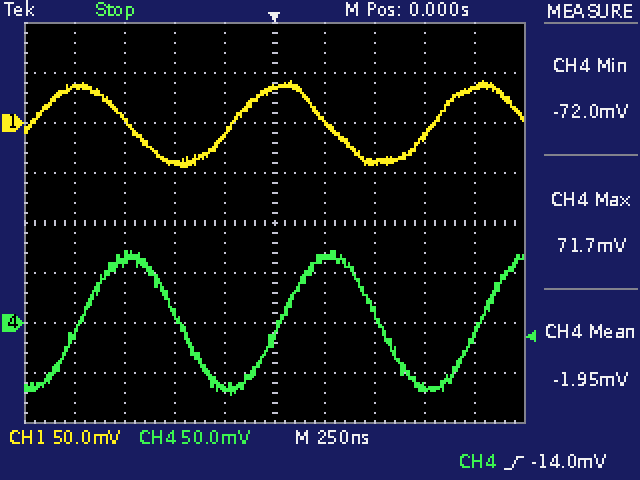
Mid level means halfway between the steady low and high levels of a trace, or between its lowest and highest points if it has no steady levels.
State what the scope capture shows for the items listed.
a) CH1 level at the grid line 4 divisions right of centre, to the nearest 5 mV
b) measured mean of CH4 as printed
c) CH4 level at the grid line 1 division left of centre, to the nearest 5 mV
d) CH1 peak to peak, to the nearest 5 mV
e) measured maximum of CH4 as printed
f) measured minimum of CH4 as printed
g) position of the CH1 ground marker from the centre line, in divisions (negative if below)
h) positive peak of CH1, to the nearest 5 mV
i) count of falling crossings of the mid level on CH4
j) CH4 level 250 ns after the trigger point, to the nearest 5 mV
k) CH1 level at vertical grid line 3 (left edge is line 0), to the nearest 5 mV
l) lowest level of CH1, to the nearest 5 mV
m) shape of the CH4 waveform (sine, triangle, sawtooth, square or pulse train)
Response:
35 mV
-1.95 mV
-65 mV
85 mV
71.7 mV
-72.0 mV
+2.0 div
40 mV
2
65 mV
-40 mV
-45 mV
sine
